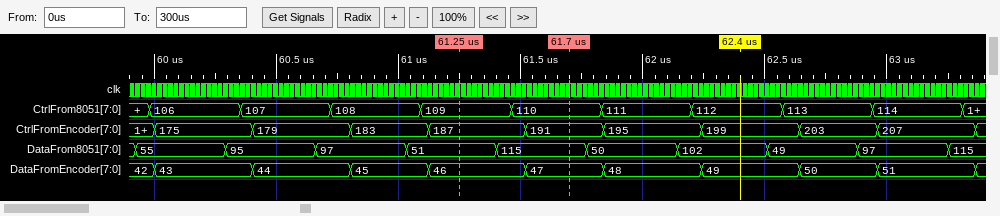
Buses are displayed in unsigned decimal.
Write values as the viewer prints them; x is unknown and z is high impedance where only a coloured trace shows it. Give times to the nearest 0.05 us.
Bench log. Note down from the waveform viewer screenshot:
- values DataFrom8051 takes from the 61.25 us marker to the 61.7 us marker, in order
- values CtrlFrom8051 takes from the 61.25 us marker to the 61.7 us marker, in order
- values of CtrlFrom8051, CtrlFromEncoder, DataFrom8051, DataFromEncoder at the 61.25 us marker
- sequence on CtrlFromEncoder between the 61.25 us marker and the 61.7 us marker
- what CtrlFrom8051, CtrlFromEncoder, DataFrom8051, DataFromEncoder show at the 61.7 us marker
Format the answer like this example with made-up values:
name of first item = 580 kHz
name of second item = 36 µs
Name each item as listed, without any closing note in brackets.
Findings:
values DataFrom8051 takes from the 61.25 us marker to the 61.7 us marker, in order = 51, 115
values CtrlFrom8051 takes from the 61.25 us marker to the 61.7 us marker, in order = 109, 110
values of CtrlFrom8051, CtrlFromEncoder, DataFrom8051, DataFromEncoder at the 61.25 us marker = CtrlFrom8051=109, CtrlFromEncoder=187, DataFrom8051=51, DataFromEncoder=46
sequence on CtrlFromEncoder between the 61.25 us marker and the 61.7 us marker = 187, 191
what CtrlFrom8051, CtrlFromEncoder, DataFrom8051, DataFromEncoder show at the 61.7 us marker = CtrlFrom8051=110, CtrlFromEncoder=191, DataFrom8051=115, DataFromEncoder=47
